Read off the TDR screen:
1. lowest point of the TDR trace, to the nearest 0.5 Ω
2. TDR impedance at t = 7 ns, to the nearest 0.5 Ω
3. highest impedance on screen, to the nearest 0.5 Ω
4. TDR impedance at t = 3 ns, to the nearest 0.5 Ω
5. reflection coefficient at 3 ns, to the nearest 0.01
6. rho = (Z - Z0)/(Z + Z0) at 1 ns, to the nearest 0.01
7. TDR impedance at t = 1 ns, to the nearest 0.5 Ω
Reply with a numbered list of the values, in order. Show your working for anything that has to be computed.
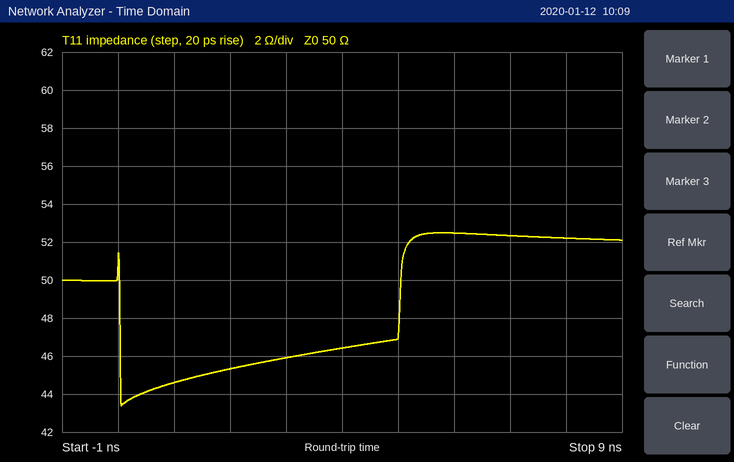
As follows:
1. 43.5 Ω
2. 52.5 Ω
3. 52.5 Ω
4. 46.0 Ω
5. (46 − 50)/(46 + 50) ≈ -0.04
6. (44.5 − 50)/(44.5 + 50) ≈ -0.06
7. 44.5 Ω
